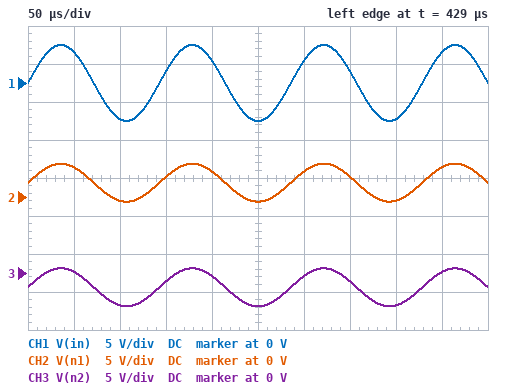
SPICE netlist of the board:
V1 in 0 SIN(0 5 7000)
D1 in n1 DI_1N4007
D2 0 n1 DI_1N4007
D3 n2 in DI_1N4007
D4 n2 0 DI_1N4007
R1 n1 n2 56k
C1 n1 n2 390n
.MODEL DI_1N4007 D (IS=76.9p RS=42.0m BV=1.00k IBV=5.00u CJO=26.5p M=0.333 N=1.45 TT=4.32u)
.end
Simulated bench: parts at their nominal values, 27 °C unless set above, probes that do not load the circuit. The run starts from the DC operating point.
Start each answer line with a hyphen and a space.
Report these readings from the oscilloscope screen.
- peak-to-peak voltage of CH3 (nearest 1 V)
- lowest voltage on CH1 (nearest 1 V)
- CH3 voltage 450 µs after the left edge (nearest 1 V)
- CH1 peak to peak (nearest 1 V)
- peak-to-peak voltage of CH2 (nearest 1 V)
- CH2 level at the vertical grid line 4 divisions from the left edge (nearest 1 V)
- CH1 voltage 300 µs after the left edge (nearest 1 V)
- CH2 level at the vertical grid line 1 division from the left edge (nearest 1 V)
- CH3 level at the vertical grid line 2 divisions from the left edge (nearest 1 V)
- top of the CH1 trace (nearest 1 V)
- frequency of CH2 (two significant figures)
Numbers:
- 5 V
- -5 V
- 0 V
- 10 V
- 5 V
- 3 V
- 3 V
- 4 V
- -4 V
- 5 V
- 7.0 kHz
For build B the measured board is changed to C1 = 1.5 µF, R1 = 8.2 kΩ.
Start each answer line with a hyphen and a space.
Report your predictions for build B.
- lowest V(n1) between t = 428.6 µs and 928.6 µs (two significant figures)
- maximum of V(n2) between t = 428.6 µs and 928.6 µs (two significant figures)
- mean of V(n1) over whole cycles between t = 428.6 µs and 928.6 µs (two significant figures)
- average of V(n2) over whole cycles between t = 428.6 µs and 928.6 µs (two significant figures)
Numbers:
- -680 mV
- 680 mV
- 1.8 V
- -1.8 V
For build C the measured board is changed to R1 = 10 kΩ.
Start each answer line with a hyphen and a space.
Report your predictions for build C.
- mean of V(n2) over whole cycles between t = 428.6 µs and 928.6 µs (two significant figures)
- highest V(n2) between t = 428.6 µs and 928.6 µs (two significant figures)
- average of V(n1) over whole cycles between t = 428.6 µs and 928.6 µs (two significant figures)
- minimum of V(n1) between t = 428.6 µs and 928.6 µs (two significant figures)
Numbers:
- -1.8 V
- 660 mV
- 1.8 V
- -660 mV
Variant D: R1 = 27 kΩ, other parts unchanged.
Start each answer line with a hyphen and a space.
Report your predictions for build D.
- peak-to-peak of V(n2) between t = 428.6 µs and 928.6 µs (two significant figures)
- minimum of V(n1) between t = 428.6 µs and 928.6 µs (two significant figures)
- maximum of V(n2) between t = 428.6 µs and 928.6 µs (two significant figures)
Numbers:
- 5.0 V
- -630 mV
- 630 mV
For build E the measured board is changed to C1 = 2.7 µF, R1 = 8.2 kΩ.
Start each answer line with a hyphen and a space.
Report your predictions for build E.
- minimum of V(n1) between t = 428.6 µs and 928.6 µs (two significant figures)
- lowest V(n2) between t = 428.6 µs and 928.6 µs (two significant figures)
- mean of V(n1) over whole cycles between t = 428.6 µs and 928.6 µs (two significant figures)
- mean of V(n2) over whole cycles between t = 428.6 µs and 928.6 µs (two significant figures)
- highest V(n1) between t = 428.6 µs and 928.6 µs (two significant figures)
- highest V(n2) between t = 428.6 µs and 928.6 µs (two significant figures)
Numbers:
- -690 mV
- -4.3 V
- 1.8 V
- -1.8 V
- 4.3 V
- 690 mV
